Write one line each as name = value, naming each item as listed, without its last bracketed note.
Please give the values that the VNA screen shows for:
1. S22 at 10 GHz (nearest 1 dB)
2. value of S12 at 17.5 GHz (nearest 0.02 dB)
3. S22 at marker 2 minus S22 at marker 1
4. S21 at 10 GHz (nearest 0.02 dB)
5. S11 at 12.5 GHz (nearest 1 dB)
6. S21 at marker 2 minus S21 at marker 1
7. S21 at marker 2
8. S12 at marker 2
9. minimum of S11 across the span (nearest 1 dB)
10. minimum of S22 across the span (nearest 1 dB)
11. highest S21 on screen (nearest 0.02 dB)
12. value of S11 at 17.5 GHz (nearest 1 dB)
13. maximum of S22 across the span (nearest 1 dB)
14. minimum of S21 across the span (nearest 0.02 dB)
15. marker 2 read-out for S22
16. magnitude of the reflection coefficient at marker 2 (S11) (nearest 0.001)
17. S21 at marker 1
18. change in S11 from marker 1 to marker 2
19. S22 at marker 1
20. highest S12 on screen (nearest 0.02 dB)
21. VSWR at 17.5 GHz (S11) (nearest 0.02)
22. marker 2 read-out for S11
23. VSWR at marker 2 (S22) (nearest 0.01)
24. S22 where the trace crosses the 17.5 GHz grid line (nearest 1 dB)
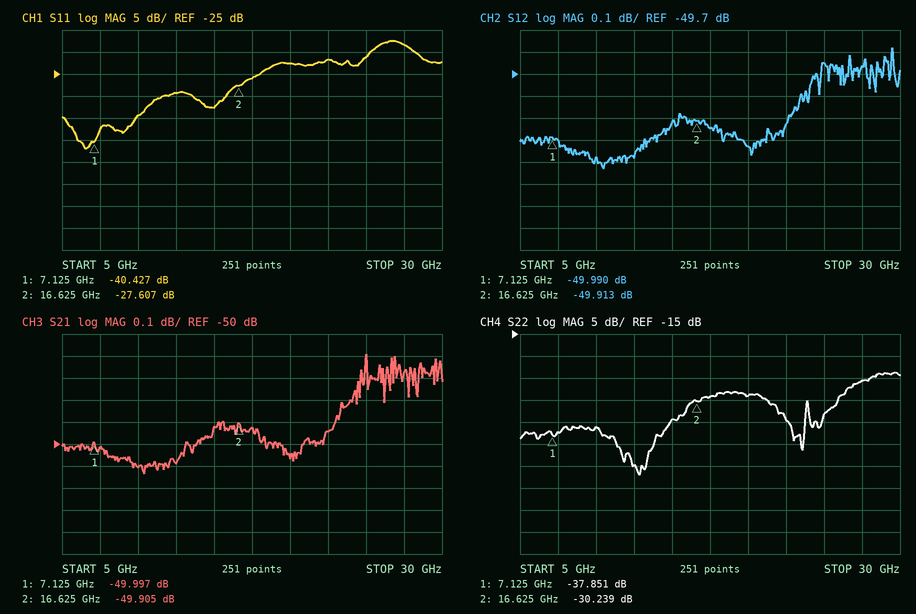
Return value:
S22 at 10 GHz = -36 dB
value of S12 at 17.5 GHz = -49.94 dB
S22 at marker 2 minus S22 at marker 1 = 7.612 dB
S21 at 10 GHz = -50.10 dB
S11 at 12.5 GHz = -29 dB
S21 at marker 2 minus S21 at marker 1 = 0.092 dB
S21 at marker 2 = -49.905 dB
S12 at marker 2 = -49.913 dB
minimum of S11 across the span = -42 dB
minimum of S22 across the span = -47 dB
highest S21 on screen = -49.60 dB
value of S11 at 17.5 GHz = -26 dB
maximum of S22 across the span = -24 dB
minimum of S21 across the span = -50.14 dB
marker 2 read-out for S22 = -30.239 dB
magnitude of the reflection coefficient at marker 2 (S11) = 0.042
S21 at marker 1 = -49.997 dB
change in S11 from marker 1 to marker 2 = 12.820 dB
S22 at marker 1 = -37.851 dB
highest S12 on screen = -49.58 dB
VSWR at 17.5 GHz (S11) = 1.10
marker 2 read-out for S11 = -27.607 dB
VSWR at marker 2 (S22) = 1.06
S22 where the trace crosses the 17.5 GHz grid line = -29 dB
